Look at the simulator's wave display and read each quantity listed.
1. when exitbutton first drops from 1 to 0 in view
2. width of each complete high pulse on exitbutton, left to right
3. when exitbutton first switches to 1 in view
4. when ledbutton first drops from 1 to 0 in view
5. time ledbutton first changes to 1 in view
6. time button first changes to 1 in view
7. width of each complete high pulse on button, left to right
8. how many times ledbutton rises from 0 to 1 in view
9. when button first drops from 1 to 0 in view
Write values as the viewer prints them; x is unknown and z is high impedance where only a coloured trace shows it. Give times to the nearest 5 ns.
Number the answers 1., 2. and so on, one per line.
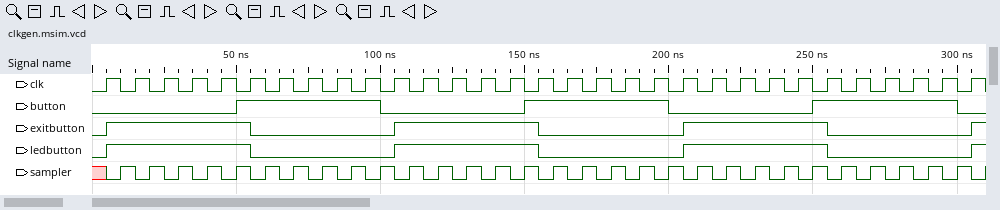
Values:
1. 55 ns
2. 50 ns, 50 ns, 50 ns
3. 5 ns
4. 55 ns
5. 5 ns
6. 50 ns
7. 50 ns, 50 ns, 50 ns
8. 4
9. 100 ns
